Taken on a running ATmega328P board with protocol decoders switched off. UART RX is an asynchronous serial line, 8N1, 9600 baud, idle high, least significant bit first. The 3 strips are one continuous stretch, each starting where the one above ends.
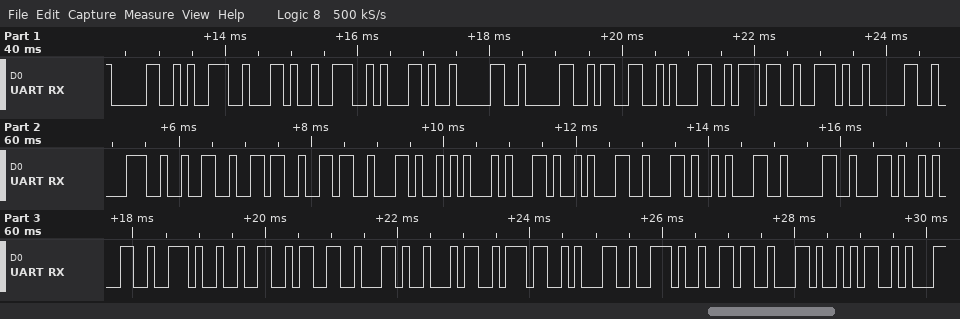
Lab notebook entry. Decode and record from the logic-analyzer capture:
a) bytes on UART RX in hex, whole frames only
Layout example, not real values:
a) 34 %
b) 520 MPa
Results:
a) 30 39 2C 4E 2C 30 30 33 31 37 2E 30 38 32 36 36 2C 45 2C 31 2C 31 30 2C 31 2E 32 33 2C 34 37 31 2E 36 2C 4D
